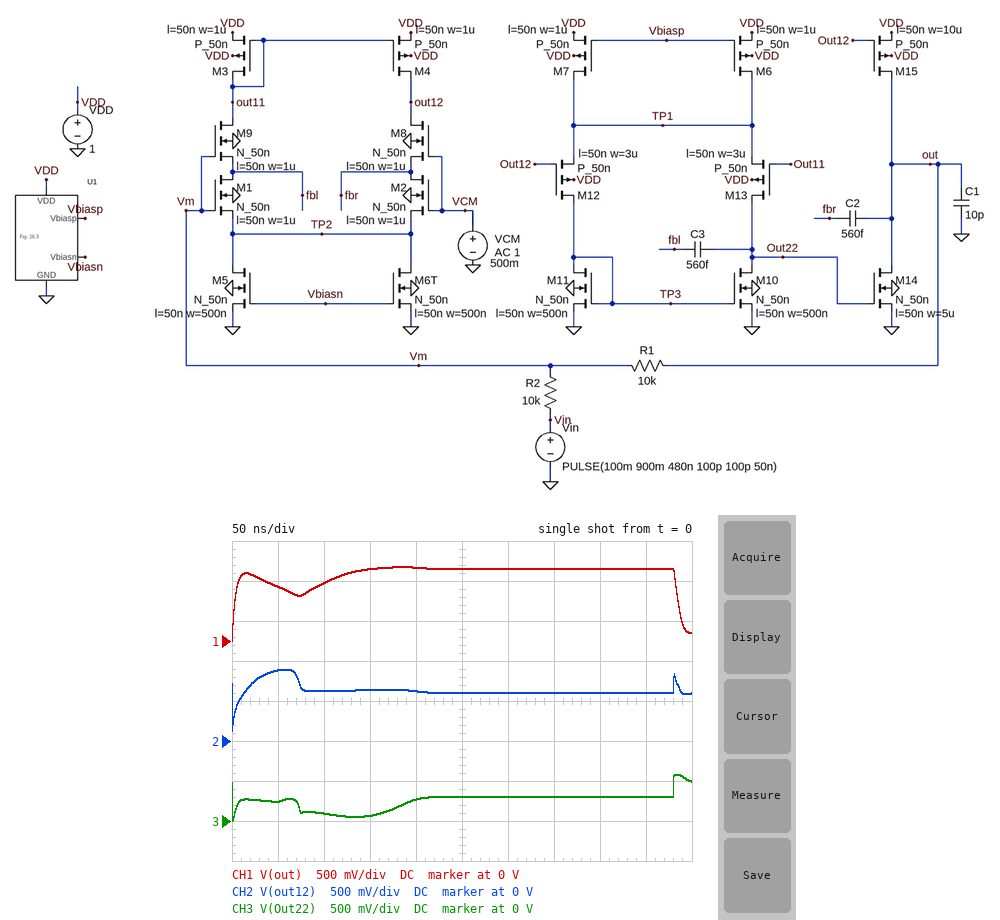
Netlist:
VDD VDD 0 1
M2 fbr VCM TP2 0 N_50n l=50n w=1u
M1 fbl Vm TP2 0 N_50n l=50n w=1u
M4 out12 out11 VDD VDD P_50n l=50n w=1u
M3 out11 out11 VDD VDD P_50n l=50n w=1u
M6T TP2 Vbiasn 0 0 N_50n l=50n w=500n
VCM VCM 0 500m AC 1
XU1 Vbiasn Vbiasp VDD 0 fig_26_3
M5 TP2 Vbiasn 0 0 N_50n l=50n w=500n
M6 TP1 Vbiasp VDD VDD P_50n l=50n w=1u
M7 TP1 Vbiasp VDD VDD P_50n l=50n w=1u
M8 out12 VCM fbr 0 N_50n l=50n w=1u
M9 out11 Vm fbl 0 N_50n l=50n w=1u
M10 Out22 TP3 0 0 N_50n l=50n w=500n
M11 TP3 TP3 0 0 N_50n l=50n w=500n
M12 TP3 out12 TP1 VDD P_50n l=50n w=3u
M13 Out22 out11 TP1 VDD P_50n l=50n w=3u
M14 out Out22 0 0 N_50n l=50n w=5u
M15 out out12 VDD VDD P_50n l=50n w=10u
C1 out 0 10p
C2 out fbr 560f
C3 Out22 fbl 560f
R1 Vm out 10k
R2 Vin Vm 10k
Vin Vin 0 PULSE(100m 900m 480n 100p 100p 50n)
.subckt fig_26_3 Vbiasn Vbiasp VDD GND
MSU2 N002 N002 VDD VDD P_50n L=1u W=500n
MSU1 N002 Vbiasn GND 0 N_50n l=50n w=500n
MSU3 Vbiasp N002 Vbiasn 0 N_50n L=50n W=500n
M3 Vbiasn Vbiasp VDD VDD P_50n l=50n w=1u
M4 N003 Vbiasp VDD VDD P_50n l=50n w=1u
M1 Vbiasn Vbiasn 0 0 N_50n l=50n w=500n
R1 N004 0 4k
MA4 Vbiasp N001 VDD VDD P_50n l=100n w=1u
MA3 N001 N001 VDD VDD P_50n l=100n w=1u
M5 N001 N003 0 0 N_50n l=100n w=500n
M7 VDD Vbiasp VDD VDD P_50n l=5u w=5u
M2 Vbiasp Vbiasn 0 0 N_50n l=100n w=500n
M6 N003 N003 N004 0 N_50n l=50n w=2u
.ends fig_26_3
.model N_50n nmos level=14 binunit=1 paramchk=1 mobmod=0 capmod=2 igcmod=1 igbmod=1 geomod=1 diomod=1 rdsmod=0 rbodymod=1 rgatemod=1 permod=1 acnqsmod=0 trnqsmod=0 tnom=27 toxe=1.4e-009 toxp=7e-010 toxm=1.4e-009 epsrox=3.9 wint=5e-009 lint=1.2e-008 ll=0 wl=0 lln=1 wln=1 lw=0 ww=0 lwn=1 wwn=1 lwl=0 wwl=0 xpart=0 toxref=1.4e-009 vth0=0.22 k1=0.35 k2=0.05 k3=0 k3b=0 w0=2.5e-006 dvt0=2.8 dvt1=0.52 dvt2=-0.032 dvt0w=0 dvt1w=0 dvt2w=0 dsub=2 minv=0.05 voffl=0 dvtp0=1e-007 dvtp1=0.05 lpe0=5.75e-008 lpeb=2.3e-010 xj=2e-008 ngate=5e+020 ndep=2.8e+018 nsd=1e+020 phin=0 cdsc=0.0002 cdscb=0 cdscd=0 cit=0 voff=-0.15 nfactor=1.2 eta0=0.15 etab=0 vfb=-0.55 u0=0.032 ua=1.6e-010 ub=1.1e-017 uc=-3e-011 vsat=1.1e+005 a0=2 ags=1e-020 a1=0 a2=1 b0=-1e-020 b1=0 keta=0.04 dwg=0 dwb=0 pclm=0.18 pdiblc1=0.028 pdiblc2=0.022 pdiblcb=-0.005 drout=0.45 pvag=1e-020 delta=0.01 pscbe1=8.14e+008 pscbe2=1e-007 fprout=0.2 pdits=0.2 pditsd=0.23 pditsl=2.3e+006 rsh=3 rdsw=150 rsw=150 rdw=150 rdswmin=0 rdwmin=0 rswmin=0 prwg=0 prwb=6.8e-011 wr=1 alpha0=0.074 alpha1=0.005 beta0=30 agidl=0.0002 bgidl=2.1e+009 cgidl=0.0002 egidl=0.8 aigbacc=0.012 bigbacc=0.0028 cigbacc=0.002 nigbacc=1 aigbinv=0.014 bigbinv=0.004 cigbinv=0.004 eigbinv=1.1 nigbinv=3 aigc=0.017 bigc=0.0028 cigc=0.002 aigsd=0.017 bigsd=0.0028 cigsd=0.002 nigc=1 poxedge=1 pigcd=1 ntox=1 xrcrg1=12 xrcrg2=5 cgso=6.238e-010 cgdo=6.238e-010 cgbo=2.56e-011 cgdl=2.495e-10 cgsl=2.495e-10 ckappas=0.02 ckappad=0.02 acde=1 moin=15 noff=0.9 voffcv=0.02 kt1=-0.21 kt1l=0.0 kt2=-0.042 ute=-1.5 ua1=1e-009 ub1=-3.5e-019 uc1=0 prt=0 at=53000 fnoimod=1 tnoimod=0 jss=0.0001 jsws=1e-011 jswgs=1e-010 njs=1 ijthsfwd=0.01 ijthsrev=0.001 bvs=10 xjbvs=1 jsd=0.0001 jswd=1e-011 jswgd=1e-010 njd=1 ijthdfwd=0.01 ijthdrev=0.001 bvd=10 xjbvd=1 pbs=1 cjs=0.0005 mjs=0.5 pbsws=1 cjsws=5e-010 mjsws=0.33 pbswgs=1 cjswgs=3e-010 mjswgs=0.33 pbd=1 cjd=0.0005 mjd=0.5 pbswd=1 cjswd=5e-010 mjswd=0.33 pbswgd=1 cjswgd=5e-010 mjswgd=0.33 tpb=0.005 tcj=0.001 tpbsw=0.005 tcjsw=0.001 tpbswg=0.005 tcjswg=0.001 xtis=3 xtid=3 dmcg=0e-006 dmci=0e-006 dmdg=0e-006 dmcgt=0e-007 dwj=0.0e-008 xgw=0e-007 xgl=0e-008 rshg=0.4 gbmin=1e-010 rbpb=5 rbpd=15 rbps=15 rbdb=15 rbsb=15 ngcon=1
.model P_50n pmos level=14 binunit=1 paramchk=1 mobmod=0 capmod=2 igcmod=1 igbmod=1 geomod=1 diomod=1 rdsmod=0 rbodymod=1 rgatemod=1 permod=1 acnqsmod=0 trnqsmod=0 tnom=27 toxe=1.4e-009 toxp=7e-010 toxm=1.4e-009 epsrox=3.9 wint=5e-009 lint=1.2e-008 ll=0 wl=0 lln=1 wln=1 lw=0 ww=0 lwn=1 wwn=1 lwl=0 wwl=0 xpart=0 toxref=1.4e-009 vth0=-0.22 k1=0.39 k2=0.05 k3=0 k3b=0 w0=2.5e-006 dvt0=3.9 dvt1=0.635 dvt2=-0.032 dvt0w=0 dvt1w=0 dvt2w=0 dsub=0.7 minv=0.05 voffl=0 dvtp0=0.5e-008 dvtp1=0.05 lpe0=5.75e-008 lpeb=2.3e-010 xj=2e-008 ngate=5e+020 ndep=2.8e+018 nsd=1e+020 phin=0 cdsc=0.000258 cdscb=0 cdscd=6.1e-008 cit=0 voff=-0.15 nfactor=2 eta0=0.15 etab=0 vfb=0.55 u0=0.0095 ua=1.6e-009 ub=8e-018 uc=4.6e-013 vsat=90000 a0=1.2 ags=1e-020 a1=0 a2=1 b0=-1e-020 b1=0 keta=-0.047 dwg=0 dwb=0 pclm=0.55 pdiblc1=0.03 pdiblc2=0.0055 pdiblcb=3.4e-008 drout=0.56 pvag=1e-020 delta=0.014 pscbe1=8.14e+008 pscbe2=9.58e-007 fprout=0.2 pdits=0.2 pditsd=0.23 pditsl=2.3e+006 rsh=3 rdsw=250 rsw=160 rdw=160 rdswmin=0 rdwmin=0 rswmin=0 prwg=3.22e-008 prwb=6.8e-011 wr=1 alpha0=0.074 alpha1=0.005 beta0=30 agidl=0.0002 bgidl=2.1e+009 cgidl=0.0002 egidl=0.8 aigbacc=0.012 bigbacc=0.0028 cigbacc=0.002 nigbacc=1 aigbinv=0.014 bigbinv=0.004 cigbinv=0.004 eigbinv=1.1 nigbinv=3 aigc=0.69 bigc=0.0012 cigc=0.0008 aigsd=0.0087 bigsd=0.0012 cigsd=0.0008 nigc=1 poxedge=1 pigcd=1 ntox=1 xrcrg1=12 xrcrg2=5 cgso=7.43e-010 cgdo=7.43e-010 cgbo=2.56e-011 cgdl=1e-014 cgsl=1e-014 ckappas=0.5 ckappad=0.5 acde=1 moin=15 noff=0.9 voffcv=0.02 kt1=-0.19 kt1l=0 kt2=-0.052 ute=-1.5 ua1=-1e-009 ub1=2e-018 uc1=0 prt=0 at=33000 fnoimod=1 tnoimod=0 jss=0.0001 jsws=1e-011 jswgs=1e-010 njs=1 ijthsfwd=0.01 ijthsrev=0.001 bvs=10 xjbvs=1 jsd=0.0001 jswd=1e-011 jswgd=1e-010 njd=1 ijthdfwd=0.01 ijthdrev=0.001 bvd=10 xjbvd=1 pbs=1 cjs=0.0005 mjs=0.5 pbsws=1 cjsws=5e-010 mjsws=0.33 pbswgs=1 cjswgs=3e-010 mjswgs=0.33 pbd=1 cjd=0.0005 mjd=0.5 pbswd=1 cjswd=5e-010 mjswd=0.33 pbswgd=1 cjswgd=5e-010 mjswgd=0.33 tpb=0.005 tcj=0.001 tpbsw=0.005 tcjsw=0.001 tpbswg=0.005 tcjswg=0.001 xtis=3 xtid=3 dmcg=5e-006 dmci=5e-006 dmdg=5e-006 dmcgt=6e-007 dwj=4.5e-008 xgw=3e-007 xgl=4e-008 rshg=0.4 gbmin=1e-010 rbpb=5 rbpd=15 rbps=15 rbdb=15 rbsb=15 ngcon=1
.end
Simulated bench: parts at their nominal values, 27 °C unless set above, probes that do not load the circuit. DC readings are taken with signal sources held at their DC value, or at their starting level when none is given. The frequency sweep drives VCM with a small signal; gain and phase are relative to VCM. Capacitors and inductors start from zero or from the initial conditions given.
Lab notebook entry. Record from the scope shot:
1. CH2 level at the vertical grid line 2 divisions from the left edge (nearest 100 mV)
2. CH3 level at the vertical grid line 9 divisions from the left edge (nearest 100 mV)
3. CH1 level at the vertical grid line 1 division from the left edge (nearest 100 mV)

600 mV
300 mV
700 mV
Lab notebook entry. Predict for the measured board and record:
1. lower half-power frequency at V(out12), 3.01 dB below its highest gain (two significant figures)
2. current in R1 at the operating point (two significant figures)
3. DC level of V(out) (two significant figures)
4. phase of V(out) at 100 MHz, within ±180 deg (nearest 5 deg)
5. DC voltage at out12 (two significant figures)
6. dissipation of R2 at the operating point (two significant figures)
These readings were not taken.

53 MHz
40 µA
900 mV
-75 deg
600 mV
16 µW
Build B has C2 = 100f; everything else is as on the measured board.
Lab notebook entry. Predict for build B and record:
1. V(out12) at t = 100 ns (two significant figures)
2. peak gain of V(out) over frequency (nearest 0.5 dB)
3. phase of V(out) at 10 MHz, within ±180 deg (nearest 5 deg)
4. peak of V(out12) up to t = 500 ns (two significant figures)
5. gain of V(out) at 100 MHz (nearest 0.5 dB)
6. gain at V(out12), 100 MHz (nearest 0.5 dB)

650 mV
6.5 dB
-15 deg
960 mV
-5.0 dB
7.5 dB
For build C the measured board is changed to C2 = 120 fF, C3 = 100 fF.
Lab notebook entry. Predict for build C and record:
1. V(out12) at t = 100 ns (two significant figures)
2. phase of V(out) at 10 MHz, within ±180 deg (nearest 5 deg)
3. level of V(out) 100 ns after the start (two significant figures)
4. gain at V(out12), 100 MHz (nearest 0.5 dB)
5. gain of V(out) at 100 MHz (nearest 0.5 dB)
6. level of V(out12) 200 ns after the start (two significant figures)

650 mV
-5 deg
890 mV
10.0 dB
1.5 dB
600 mV
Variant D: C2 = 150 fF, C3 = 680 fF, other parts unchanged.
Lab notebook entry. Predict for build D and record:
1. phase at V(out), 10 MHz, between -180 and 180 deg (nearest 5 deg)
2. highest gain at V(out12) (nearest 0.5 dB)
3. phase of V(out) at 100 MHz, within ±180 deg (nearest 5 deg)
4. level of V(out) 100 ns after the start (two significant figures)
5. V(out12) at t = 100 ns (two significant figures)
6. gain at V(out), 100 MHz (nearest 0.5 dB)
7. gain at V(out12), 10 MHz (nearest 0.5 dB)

-15 deg
7.0 dB
-90 deg
880 mV
650 mV
-5.5 dB
-4.0 dB
